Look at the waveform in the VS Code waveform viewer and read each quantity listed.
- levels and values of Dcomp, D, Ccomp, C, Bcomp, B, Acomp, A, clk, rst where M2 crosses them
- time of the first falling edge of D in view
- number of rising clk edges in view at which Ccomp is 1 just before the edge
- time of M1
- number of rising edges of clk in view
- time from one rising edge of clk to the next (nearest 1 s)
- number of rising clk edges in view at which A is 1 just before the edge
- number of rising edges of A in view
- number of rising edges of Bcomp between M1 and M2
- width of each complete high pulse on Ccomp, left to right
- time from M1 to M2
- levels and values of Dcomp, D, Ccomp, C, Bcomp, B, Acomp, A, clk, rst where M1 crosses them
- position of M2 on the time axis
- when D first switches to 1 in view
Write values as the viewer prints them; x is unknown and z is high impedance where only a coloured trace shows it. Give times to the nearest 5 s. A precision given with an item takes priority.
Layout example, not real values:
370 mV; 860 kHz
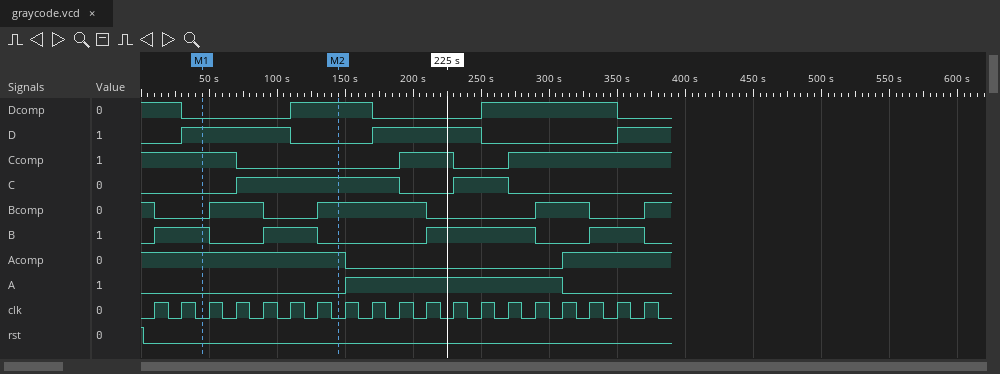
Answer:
Dcomp=1, D=0, Ccomp=0, C=1, Bcomp=1, B=0, Acomp=1, A=0, clk=0, rst=0; 110 s; 11; 45 s; 19; 20 s; 8; 1; 2; 40 s; 100 s; Dcomp=0, D=1, Ccomp=1, C=0, Bcomp=0, B=1, Acomp=1, A=0, clk=0, rst=0; 145 s; 30 s
